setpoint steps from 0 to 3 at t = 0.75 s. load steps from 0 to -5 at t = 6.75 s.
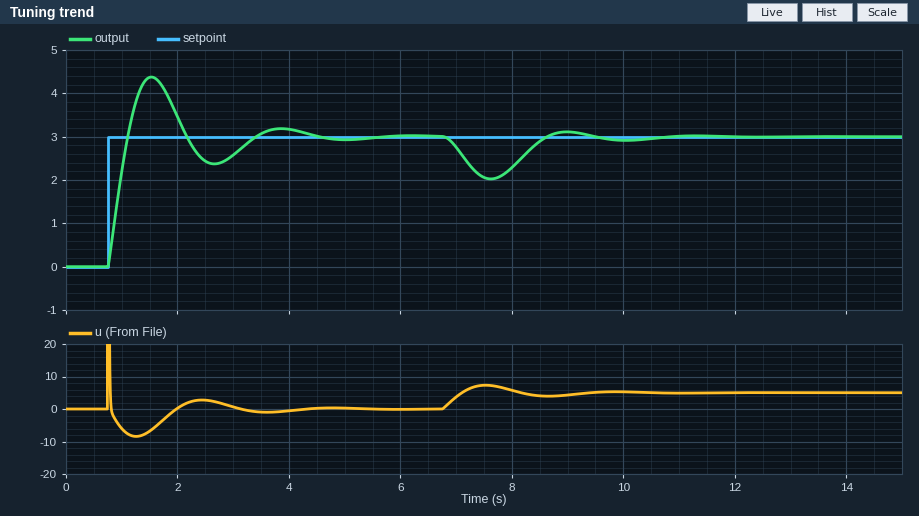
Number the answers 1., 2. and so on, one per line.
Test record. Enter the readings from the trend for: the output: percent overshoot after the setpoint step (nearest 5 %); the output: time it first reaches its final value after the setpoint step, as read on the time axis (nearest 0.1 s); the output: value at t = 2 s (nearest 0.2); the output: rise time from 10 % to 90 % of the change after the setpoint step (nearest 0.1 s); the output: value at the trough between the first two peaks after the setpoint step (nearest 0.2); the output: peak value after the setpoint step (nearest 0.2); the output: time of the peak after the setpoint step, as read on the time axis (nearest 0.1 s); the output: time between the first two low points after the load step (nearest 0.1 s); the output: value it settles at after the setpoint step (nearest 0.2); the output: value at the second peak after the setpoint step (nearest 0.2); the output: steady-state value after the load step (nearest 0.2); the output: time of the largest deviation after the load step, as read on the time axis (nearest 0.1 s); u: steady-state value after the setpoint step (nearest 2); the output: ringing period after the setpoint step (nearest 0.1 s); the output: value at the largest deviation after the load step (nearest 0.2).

1. 45 %
2. 1.1 s
3. 3.4
4. 0.3 s
5. 2.4
6. 4.4
7. 1.5 s
8. 2.4 s
9. 3.0
10. 3.2
11. 3.0
12. 7.6 s
13. 0
14. 2.3 s
15. 2.0
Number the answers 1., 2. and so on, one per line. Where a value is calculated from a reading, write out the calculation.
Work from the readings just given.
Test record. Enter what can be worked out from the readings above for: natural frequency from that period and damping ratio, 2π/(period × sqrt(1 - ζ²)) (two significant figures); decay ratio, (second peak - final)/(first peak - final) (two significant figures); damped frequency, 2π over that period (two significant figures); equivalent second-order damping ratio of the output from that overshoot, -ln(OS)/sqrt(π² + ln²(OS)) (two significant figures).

1. 2π / (2.3 × sqrt(1 - 0.25²)) = 2.8 rad/s
2. (3.2 - 3) / (4.4 - 3) = 0.14
3. 2π / 2.3 = 2.7 rad/s
4. ln(0.45) = -0.799; 0.799 / sqrt(9.870 + 0.638) = 0.25
